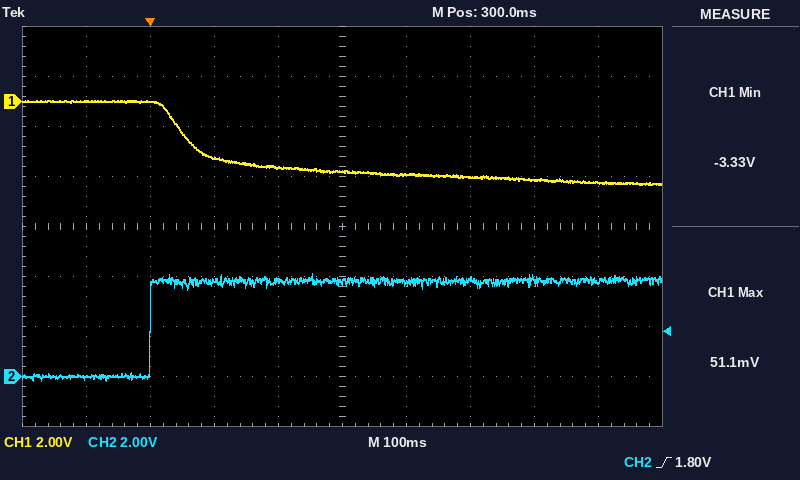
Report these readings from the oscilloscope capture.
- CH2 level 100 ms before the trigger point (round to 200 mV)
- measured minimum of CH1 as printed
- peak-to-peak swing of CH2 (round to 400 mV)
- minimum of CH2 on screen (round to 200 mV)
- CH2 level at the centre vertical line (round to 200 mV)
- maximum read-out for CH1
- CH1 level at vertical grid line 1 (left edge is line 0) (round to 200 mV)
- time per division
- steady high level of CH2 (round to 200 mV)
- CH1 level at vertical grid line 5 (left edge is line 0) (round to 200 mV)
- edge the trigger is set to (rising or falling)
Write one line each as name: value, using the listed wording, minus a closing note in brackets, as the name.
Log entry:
CH2 level 100 ms before the trigger point: 0.0 V
measured minimum of CH1 as printed: -3.33 V
peak-to-peak swing of CH2: 4.4 V
minimum of CH2 on screen: -200 mV
CH2 level at the centre vertical line: 3.8 V
maximum read-out for CH1: 51.1 mV
CH1 level at vertical grid line 1 (left edge is line 0): 0.0 V
time per division: 100 ms
steady high level of CH2: 3.8 V
CH1 level at vertical grid line 5 (left edge is line 0): -2.8 V
edge the trigger is set to: rising
